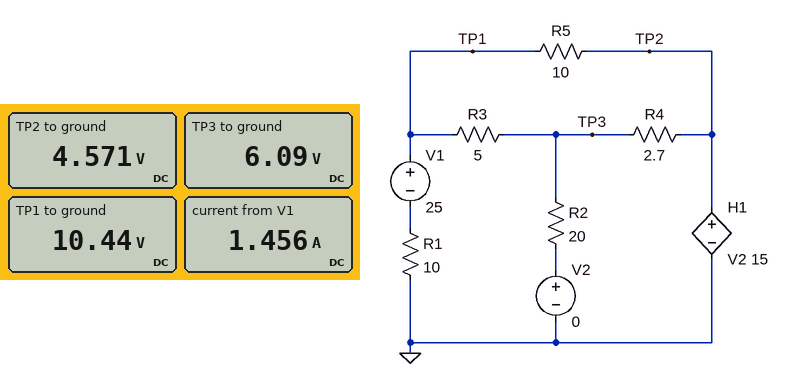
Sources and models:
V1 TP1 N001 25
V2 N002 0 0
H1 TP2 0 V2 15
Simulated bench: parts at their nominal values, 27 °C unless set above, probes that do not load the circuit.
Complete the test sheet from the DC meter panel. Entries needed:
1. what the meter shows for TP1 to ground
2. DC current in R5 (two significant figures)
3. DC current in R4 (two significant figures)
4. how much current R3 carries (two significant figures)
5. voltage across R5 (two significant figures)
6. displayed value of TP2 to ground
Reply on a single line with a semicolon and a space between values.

10.44 V; 590 mA; 560 mA; 870 mA; 5.9 V; 4.571 V
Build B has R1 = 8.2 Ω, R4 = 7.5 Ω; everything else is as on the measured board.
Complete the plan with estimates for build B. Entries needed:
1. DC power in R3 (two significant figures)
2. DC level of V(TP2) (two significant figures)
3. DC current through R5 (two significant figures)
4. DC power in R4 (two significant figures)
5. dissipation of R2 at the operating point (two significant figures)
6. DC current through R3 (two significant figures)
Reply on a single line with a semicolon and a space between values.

3.1 W; 7.1 V; 630 mA; 740 mW; 4.5 W; 790 mA
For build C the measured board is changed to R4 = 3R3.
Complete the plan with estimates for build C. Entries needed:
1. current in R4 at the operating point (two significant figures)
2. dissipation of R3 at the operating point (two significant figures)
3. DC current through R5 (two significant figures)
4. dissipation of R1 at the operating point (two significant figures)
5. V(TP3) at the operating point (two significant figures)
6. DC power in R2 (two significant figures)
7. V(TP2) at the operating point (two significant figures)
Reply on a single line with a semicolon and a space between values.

500 mA; 3.5 W; 580 mA; 20 W; 6.6 V; 2.2 W; 5.0 V
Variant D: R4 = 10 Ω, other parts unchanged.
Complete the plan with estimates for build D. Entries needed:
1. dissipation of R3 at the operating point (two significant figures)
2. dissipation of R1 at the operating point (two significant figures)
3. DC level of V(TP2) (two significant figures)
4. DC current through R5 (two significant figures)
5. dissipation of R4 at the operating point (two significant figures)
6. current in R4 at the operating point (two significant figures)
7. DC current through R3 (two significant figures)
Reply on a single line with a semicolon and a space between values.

2.3 W; 16 W; 6.8 V; 570 mA; 520 mW; 230 mA; 680 mA
